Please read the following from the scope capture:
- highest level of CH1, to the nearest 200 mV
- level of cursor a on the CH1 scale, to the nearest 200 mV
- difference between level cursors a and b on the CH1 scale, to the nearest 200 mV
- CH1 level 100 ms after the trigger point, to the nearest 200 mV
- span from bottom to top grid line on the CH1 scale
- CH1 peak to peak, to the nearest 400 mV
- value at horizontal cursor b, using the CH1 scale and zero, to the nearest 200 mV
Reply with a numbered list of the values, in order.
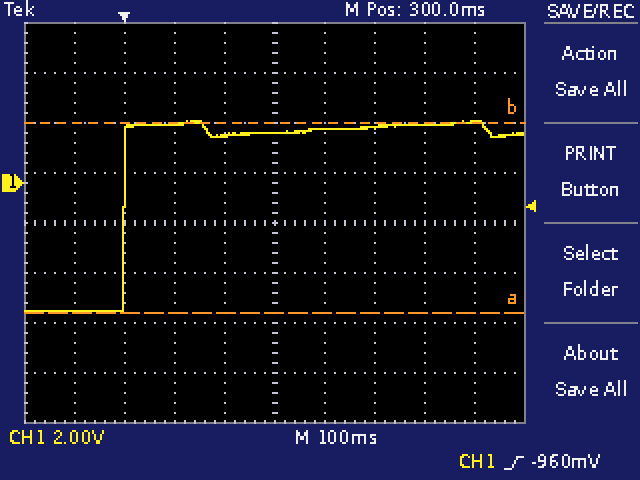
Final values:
1. 2.4 V
2. -5.2 V
3. 7.6 V
4. 2.4 V
5. 16 V
6. 7.6 V
7. 2.4 V
